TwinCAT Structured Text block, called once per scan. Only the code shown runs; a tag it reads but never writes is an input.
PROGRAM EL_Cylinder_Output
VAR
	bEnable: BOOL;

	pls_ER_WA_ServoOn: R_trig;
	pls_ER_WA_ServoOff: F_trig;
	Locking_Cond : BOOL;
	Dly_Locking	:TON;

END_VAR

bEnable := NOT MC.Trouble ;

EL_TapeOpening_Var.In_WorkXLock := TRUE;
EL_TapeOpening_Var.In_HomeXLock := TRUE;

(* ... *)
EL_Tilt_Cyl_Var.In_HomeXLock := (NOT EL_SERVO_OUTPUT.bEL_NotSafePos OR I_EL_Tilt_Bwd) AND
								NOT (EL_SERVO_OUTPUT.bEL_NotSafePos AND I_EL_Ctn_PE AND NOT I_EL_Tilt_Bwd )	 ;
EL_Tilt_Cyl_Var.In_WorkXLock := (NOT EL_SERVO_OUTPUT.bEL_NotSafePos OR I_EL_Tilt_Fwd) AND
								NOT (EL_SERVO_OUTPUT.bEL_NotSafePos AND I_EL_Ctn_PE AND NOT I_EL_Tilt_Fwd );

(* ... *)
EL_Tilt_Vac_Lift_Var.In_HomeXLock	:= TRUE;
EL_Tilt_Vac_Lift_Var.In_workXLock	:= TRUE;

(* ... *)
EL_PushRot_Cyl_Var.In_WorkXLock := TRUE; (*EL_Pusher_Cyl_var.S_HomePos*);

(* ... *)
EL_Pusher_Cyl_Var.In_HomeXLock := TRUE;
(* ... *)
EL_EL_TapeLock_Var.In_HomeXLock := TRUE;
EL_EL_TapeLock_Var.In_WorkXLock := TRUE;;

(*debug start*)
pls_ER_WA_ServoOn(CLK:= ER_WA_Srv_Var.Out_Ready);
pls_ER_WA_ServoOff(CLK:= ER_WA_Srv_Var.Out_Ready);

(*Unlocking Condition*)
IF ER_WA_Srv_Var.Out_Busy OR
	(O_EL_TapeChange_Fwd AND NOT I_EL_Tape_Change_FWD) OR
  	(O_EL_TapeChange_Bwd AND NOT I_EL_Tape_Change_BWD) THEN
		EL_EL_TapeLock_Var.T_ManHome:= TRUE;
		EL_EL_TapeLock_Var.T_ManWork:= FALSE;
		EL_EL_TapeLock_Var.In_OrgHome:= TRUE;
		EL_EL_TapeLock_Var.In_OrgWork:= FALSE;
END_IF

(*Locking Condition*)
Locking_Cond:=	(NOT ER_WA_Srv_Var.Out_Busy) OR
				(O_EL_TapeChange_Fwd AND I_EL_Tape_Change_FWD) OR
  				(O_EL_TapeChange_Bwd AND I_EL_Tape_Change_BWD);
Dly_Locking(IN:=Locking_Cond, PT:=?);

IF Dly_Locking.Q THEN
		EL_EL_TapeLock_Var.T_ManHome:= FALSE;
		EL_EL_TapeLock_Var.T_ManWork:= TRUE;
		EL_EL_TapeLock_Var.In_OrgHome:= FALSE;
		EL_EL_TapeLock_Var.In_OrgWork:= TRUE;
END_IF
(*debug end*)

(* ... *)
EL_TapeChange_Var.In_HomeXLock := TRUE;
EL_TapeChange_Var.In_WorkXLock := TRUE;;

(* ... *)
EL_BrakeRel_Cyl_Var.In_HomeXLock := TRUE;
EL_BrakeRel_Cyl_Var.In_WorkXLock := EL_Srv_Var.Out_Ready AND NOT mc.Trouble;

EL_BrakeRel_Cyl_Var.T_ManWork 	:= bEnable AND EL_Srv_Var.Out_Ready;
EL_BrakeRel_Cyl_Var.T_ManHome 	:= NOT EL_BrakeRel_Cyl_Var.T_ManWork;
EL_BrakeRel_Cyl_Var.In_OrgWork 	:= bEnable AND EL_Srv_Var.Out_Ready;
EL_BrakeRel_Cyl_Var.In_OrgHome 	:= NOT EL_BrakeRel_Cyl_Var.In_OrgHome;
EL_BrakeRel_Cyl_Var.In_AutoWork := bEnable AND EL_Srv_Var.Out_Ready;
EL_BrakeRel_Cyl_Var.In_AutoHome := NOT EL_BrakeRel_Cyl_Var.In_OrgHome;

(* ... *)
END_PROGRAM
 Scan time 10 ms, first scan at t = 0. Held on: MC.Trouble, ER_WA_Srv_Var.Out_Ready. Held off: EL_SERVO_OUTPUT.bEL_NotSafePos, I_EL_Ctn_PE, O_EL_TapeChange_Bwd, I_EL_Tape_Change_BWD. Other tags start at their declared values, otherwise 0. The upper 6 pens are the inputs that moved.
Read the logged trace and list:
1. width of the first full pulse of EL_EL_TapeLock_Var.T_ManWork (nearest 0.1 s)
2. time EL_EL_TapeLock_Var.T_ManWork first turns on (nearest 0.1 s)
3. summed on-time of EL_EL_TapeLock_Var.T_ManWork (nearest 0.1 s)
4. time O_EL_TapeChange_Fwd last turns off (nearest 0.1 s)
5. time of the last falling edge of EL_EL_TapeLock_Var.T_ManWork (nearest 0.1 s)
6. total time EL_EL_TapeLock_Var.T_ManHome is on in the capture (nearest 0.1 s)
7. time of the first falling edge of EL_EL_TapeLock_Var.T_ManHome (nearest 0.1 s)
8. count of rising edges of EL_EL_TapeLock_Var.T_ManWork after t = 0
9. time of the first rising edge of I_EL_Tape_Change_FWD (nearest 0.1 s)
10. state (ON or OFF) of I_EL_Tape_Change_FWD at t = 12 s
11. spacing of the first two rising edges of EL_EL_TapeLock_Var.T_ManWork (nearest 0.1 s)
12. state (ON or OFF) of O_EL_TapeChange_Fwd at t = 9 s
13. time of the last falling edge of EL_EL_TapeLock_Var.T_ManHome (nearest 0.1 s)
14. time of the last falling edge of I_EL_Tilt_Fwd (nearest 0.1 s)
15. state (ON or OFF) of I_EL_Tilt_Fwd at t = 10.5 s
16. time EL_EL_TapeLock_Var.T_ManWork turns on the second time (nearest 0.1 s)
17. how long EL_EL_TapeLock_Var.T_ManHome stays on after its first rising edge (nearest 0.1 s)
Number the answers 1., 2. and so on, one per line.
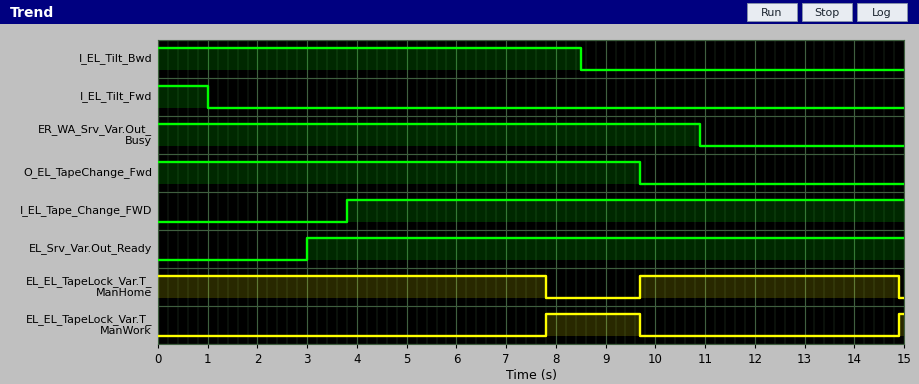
1. 1.9 s
2. 7.8 s
3. 2.0 s
4. 9.7 s
5. 9.7 s
6. 13.0 s
7. 7.8 s
8. 2
9. 3.8 s
10. ON
11. 7.1 s
12. ON
13. 14.9 s
14. 1.0 s
15. OFF
16. 14.9 s
17. 5.2 s
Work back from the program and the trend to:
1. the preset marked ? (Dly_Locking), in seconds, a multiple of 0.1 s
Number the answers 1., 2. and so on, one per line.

1. 4.0 s
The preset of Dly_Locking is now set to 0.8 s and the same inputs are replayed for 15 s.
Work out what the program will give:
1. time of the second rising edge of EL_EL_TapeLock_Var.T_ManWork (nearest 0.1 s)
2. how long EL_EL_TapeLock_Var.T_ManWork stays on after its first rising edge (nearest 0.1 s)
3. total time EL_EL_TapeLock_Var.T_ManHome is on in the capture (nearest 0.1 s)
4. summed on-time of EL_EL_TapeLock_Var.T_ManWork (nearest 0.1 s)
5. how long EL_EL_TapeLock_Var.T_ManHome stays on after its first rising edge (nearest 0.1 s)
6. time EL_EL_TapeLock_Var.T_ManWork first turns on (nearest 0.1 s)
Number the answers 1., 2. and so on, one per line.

1. 11.7 s
2. 5.1 s
3. 6.6 s
4. 8.4 s
5. 2.0 s
6. 4.6 s
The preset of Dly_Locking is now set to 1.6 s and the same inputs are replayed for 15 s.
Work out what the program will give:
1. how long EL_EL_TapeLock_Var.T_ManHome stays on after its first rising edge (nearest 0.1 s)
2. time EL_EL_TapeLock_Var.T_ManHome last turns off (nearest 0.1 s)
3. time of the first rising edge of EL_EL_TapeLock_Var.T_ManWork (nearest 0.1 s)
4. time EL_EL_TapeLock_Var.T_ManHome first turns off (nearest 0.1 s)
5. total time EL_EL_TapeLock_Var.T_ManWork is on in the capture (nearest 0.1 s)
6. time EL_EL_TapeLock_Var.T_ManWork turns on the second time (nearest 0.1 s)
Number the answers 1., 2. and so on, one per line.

1. 2.8 s
2. 12.5 s
3. 5.4 s
4. 5.4 s
5. 6.8 s
6. 12.5 s
